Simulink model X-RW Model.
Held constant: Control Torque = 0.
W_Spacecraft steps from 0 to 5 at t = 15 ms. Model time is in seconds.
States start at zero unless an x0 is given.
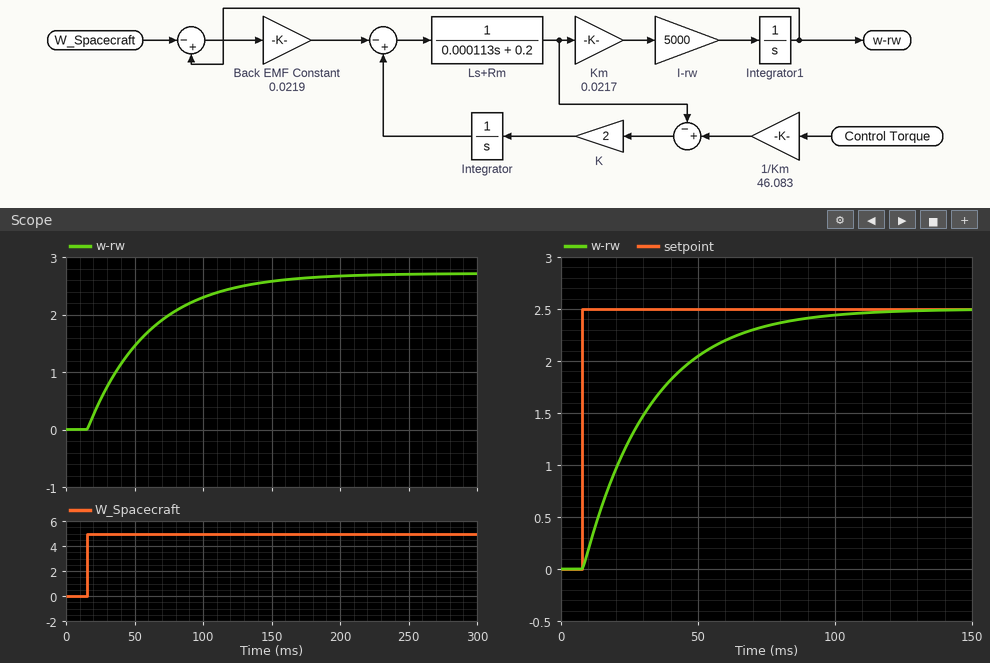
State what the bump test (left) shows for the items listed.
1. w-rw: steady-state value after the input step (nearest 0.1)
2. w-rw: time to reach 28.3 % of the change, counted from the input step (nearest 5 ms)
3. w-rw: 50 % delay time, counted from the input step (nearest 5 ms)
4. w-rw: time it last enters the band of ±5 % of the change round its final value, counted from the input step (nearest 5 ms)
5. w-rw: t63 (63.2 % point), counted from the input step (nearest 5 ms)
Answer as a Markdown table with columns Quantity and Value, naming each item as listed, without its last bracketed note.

| Quantity | Value |
|---|---|
| w-rw: steady-state value after the input step | 2.7 |
| w-rw: time to reach 28.3 % of the change, counted from the input step | 15 ms |
| w-rw: 50 % delay time, counted from the input step | 30 ms |
| w-rw: time it last enters the band of ±5 % of the change round its final value, counted from the input step | 135 ms |
| w-rw: t63 (63.2 % point), counted from the input step | 45 ms |
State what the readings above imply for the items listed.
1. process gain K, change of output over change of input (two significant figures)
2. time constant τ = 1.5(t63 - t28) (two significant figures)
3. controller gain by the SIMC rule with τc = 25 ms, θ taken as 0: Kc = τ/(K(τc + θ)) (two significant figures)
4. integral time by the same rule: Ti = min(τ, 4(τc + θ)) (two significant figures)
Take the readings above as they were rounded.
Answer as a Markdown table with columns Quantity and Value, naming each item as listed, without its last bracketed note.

| Quantity | Value |
|---|---|
| process gain K, change of output over change of input | 0.54 |
| time constant τ = 1.5(t63 - t28) | 45 ms |
| controller gain by the SIMC rule with τc = 25 ms, θ taken as 0: Kc = τ/(K(τc + θ)) | 3.3 |
| integral time by the same rule: Ti = min(τ, 4(τc + θ)) | 45 ms |
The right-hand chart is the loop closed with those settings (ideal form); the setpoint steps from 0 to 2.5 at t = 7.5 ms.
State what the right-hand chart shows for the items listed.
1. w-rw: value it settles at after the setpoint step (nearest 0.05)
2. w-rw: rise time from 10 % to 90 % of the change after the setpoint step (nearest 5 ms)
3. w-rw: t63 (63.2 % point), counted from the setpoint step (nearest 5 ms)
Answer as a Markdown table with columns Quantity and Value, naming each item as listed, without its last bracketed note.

| Quantity | Value |
|---|---|
| w-rw: value it settles at after the setpoint step | 2.50 |
| w-rw: rise time from 10 % to 90 % of the change after the setpoint step | 55 ms |
| w-rw: t63 (63.2 % point), counted from the setpoint step | 25 ms |
